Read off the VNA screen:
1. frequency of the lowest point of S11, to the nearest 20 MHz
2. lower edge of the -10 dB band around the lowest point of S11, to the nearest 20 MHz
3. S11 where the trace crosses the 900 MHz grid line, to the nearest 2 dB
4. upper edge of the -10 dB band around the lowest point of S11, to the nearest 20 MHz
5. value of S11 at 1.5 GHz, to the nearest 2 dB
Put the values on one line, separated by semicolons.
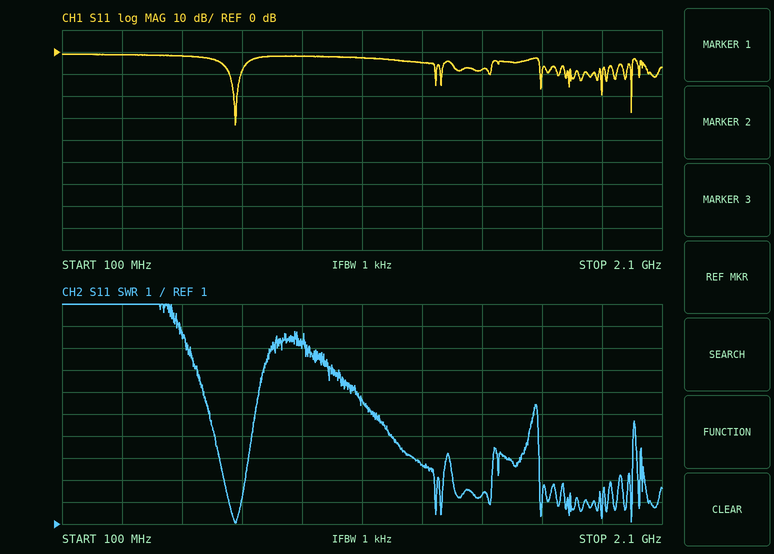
680 MHz; 660 MHz; -2 dB; 700 MHz; -8 dB
